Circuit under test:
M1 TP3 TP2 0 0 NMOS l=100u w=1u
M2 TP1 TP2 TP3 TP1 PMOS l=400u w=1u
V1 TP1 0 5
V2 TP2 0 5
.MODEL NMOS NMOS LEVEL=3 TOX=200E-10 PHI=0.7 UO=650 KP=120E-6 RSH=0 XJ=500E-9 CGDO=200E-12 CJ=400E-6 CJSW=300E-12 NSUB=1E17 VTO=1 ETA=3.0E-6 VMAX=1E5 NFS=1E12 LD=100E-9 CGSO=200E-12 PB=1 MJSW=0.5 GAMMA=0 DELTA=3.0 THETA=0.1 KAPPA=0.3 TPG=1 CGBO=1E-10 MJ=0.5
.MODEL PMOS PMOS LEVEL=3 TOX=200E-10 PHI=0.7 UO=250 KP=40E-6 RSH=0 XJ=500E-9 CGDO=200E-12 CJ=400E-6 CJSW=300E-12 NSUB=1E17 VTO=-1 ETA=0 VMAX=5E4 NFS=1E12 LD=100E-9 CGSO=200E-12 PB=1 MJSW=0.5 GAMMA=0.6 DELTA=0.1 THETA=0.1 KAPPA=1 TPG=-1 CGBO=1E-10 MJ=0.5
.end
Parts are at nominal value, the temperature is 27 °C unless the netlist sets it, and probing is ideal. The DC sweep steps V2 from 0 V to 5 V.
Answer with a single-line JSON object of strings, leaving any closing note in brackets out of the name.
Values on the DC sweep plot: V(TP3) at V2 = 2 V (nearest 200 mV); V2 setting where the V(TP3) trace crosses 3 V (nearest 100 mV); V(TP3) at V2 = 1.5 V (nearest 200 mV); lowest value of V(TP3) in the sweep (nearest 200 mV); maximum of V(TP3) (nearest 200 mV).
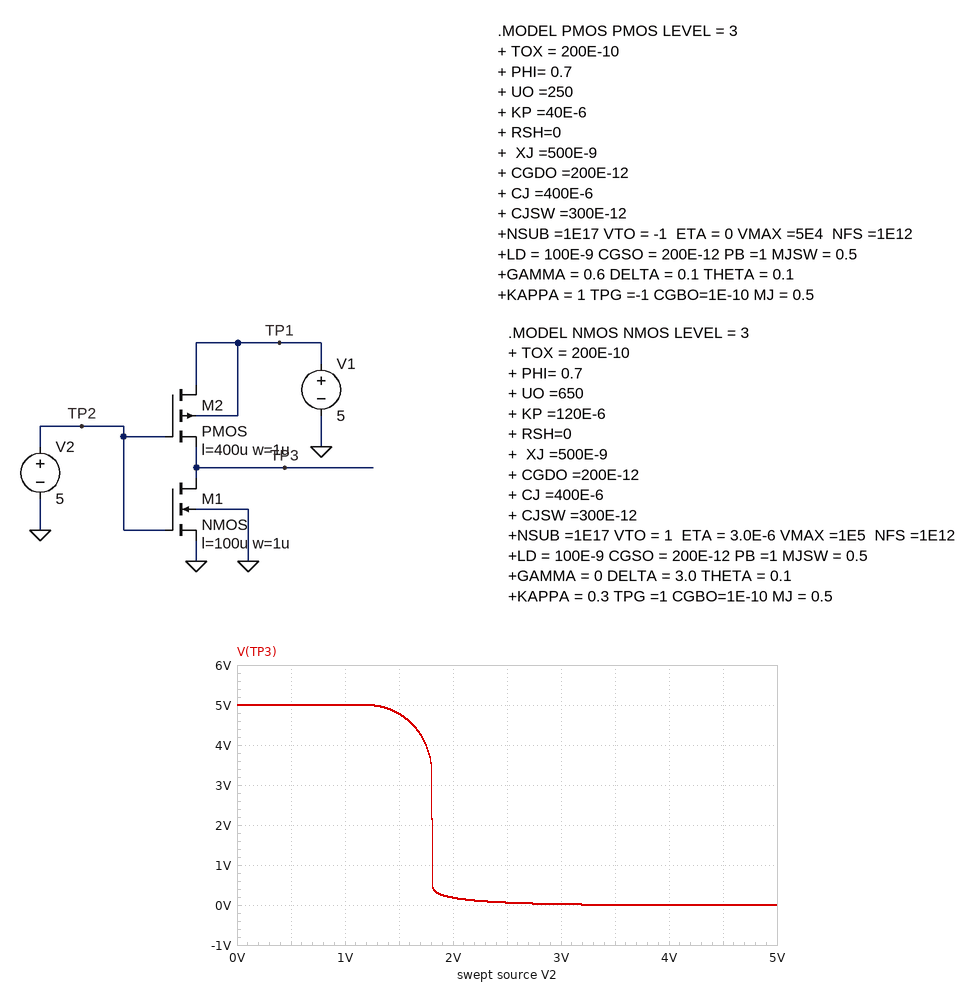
{"V(TP3) at V2 = 2 V": "200 mV", "V2 setting where the V(TP3) trace crosses 3 V": "1.8 V", "V(TP3) at V2 = 1.5 V": "4.8 V", "lowest value of V(TP3) in the sweep": "0 V", "maximum of V(TP3)": "5.0 V"}
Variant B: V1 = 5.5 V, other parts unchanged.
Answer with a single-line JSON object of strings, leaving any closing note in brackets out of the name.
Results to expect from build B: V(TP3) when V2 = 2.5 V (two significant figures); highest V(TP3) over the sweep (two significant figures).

{"V(TP3) when V2 = 2.5 V": "110 mV", "highest V(TP3) over the sweep": "5.5 V"}
